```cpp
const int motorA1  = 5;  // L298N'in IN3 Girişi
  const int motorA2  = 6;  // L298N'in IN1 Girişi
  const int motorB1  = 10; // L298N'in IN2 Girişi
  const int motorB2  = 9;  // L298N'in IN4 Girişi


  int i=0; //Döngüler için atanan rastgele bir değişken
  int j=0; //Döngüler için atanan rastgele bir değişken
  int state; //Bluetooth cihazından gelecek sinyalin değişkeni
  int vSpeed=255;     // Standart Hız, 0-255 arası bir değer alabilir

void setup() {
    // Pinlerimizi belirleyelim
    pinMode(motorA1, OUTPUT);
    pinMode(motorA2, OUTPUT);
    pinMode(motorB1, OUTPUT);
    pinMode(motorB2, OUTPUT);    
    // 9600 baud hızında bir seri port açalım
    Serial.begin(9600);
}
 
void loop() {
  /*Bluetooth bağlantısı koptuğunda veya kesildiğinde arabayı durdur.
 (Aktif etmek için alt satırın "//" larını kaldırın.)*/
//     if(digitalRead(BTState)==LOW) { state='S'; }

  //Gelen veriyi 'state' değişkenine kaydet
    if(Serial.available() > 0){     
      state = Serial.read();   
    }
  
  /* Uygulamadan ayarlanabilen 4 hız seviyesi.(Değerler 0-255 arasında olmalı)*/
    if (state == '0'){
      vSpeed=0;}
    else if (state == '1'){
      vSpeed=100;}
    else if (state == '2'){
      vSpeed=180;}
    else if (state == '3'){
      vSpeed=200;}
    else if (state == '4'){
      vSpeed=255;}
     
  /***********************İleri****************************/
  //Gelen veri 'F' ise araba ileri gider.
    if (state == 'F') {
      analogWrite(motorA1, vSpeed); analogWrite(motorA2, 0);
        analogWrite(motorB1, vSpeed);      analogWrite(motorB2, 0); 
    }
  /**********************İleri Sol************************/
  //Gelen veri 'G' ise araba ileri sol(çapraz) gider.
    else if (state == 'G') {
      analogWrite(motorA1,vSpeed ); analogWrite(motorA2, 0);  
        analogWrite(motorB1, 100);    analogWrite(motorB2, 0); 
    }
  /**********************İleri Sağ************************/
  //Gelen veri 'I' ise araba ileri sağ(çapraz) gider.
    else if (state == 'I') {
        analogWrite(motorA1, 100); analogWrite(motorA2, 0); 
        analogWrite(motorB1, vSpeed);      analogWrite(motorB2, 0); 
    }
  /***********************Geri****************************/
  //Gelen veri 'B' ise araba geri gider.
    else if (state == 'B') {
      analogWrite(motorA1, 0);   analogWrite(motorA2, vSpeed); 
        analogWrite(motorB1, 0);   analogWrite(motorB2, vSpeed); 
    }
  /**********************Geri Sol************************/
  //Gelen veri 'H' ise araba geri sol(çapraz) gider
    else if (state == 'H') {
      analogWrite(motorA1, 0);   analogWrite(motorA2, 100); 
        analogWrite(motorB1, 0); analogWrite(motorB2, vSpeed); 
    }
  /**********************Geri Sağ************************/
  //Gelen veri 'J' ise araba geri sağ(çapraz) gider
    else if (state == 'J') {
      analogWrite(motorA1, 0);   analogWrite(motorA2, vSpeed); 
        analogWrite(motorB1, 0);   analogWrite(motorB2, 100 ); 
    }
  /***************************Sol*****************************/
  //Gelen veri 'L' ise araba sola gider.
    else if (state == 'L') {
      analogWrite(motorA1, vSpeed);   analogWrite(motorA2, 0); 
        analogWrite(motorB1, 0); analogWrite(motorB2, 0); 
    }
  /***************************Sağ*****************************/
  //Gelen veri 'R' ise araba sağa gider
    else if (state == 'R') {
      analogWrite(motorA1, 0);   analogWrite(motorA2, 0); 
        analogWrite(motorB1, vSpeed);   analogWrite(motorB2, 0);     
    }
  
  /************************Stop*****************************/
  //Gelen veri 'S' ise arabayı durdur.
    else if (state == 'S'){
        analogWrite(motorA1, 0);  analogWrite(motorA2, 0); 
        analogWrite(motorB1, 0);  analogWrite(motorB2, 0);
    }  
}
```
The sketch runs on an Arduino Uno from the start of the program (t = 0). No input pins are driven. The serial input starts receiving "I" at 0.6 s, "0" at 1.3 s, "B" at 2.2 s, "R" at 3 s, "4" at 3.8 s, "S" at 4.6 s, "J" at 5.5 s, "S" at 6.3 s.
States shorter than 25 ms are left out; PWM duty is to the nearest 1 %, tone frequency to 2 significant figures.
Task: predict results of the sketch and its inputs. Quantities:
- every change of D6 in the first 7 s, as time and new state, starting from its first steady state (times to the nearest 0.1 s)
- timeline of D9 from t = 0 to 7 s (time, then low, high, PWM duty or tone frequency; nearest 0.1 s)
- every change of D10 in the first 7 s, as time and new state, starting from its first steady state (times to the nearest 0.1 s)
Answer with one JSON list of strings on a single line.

["0 s low; 5.5 s high; 6.3 s low", "0 s low; 5.5 s PWM 39 %; 6.3 s low", "0 s low; 0.6 s high; 2.2 s low"]
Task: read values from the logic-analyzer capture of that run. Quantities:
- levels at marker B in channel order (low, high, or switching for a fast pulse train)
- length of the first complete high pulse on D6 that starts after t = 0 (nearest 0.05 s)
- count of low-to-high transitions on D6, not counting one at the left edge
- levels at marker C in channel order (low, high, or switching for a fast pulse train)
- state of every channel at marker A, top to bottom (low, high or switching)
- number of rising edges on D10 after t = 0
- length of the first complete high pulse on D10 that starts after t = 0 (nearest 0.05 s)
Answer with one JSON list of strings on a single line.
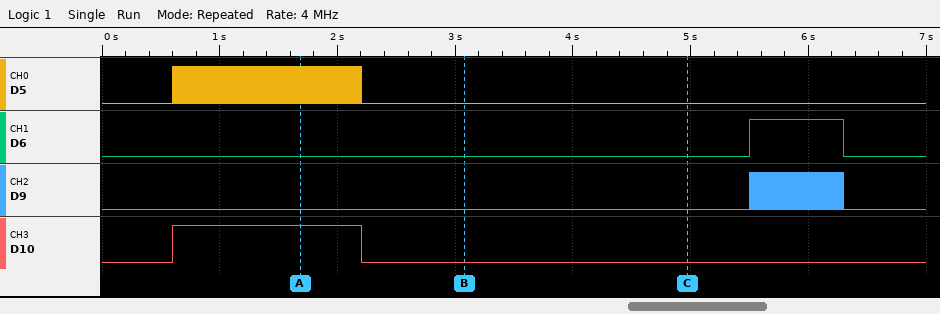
["D5 low, D6 low, D9 low, D10 low", "0.80 s", "1", "D5 low, D6 low, D9 low, D10 low", "D5 switching, D6 low, D9 low, D10 high", "1", "1.60 s"]
